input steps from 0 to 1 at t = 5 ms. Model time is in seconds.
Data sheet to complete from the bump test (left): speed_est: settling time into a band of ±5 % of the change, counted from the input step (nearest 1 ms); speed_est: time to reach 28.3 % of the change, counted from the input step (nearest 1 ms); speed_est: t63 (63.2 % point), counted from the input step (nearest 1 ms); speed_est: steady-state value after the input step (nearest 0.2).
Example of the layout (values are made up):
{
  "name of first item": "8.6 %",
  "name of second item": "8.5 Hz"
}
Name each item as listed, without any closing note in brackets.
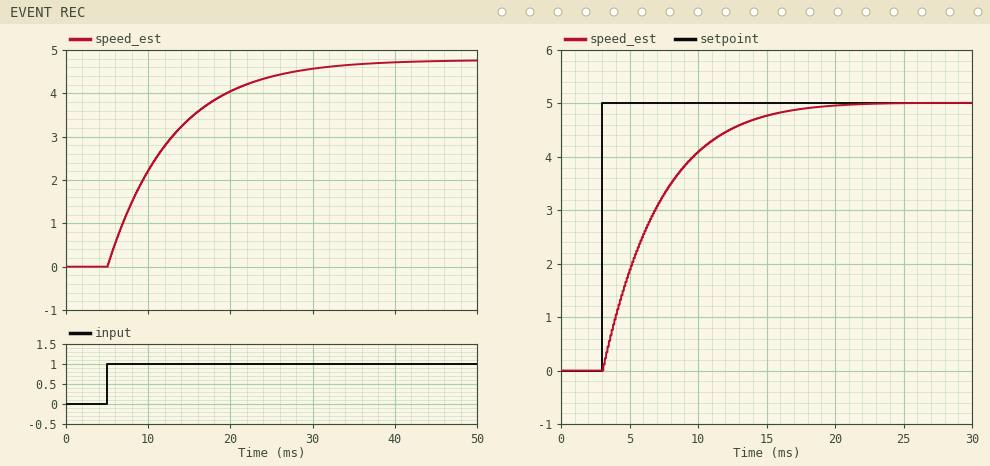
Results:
{
  "speed_est: settling time into a band of ±5 % of the change, counted from the input step": "24 ms",
  "speed_est: time to reach 28.3 % of the change, counted from the input step": "3 ms",
  "speed_est: t63 (63.2 % point), counted from the input step": "8 ms",
  "speed_est: steady-state value after the input step": "4.8"
}
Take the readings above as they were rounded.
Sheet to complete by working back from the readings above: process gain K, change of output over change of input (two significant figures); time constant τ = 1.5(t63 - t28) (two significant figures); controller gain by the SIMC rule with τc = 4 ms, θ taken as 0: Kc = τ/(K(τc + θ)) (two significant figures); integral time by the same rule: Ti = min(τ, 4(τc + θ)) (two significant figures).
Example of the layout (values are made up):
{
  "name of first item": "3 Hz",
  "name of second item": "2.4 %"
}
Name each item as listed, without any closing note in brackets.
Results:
{
  "process gain K, change of output over change of input": "4.8",
  "time constant τ = 1.5(t63 - t28)": "7.5 ms",
  "controller gain by the SIMC rule with τc = 4 ms, θ taken as 0: Kc = τ/(K(τc + θ))": "0.39",
  "integral time by the same rule: Ti = min(τ, 4(τc + θ))": "7.5 ms"
}
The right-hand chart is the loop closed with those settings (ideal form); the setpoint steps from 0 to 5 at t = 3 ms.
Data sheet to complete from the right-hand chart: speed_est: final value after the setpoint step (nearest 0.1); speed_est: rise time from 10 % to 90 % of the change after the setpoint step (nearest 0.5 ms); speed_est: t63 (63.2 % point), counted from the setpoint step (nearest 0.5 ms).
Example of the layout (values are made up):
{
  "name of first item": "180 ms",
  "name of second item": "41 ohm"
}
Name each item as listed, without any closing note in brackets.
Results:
{
  "speed_est: final value after the setpoint step": "5.0",
  "speed_est: rise time from 10 % to 90 % of the change after the setpoint step": "9.0 ms",
  "speed_est: t63 (63.2 % point), counted from the setpoint step": "4.0 ms"
}
